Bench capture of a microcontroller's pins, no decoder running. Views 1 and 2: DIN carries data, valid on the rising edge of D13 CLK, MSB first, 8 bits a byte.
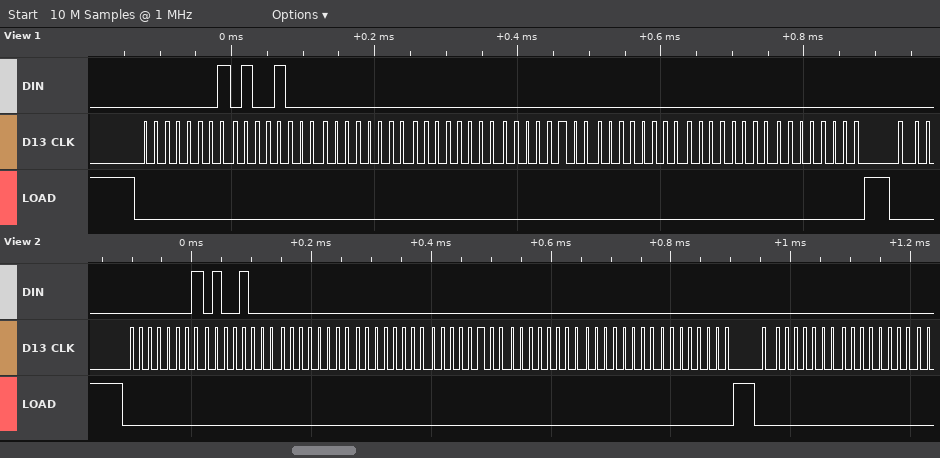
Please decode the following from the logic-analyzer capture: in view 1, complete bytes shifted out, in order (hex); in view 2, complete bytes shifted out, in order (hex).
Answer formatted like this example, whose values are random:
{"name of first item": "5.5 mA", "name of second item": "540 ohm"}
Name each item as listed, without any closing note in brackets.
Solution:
{"in view 1, complete bytes shifted out, in order": "0x01 0x48 0x00 0x00 0x00 0x00 0x00 0x00", "in view 2, complete bytes shifted out, in order": "01 48 00 00 00 00 00 00 00 00"}
